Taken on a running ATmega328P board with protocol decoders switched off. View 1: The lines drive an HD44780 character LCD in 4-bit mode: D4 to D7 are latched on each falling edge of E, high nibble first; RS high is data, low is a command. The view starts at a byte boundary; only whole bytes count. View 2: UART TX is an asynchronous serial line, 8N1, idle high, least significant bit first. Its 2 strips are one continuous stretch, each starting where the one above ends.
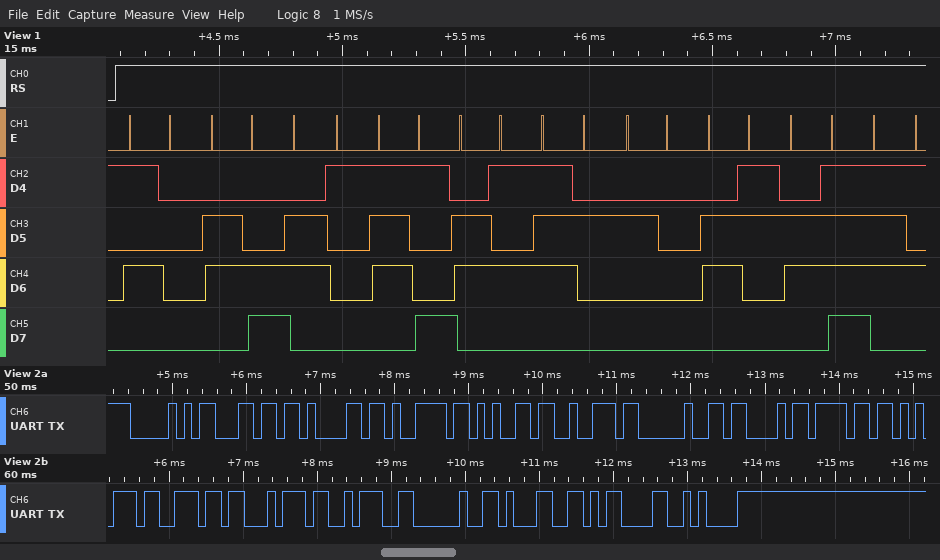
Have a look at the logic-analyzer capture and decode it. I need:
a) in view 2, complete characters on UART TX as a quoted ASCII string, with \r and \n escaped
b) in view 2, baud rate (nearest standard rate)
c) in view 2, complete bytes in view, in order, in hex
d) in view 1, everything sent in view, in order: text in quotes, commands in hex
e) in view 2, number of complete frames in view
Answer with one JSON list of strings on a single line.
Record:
["\"Player Count: 1\\r\\n\"", "9600 baud", "50 6C 61 79 65 72 20 43 6F 75 6E 74 3A 20 31 0D 0A", "\"Player cou\"", "17"]
